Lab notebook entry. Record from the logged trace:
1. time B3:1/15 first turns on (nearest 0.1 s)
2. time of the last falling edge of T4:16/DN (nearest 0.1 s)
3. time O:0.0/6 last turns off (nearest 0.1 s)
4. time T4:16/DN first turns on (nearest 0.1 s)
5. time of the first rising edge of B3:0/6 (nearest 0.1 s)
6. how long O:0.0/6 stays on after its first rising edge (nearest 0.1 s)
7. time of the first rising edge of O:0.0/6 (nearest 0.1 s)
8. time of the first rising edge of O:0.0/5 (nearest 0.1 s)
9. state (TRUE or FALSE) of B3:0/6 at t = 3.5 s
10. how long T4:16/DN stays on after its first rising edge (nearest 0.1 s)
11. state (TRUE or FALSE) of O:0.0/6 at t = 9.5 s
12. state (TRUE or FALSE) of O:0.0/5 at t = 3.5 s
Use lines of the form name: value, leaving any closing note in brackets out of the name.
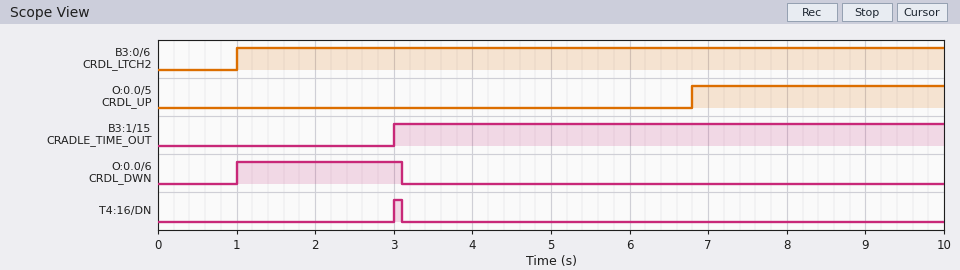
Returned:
time B3:1/15 first turns on: 3.0 s
time of the last falling edge of T4:16/DN: 3.1 s
time O:0.0/6 last turns off: 3.1 s
time T4:16/DN first turns on: 3.0 s
time of the first rising edge of B3:0/6: 1.0 s
how long O:0.0/6 stays on after its first rising edge: 2.1 s
time of the first rising edge of O:0.0/6: 1.0 s
time of the first rising edge of O:0.0/5: 6.8 s
state (TRUE or FALSE) of B3:0/6 at t = 3.5 s: TRUE
how long T4:16/DN stays on after its first rising edge: 0.1 s
state (TRUE or FALSE) of O:0.0/6 at t = 9.5 s: FALSE
state (TRUE or FALSE) of O:0.0/5 at t = 3.5 s: FALSE
